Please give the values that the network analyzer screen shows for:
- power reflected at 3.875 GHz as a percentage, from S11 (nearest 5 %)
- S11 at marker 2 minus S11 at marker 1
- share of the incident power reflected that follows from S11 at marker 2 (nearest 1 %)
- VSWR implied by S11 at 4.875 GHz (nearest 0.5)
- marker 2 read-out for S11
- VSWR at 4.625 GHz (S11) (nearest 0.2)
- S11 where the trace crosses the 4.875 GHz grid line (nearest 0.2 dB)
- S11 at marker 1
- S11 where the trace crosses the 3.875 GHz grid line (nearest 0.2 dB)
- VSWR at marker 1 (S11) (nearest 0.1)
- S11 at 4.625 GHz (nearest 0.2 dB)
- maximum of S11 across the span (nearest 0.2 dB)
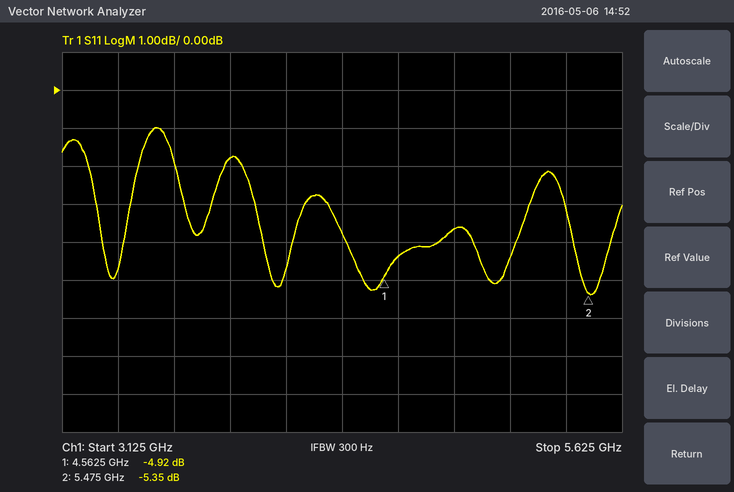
65 %
-0.43 dB
29 %
5.0
-5.35 dB
4.0
-3.6 dB
-4.92 dB
-1.8 dB
3.6
-4.4 dB
-1.0 dB
